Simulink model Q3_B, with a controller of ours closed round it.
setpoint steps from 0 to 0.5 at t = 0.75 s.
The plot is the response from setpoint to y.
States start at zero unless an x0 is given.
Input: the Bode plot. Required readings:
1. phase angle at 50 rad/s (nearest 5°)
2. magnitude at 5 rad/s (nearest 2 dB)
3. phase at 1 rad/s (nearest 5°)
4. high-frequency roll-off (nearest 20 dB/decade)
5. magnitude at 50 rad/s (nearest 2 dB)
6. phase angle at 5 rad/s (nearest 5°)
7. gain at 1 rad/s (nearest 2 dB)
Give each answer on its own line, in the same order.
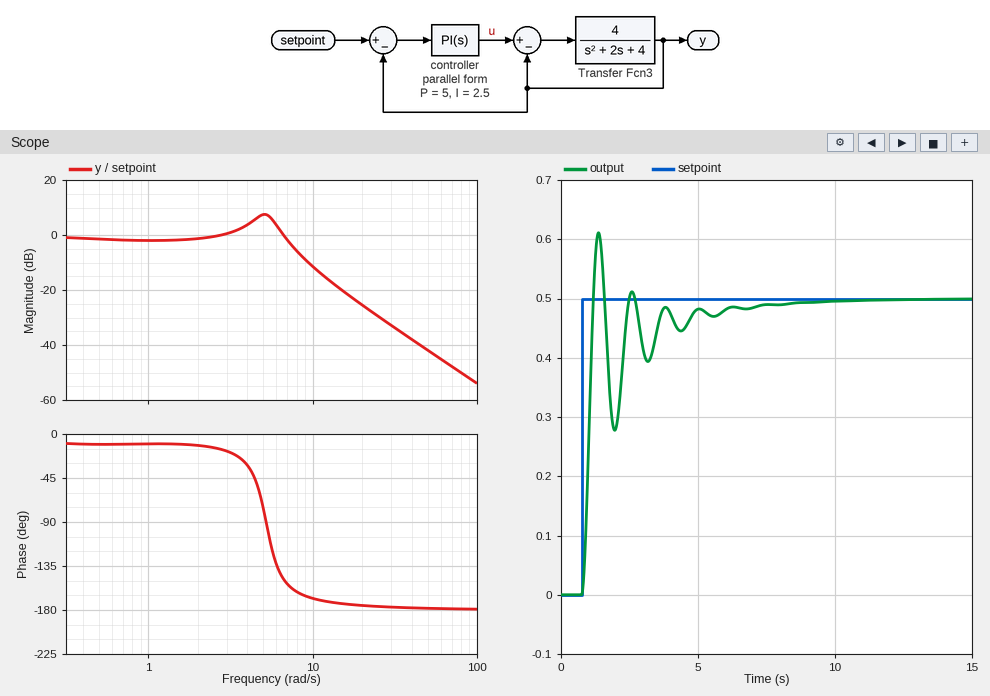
-180°
8 dB
-10°
-40 dB/decade
-42 dB
-75°
-2 dB
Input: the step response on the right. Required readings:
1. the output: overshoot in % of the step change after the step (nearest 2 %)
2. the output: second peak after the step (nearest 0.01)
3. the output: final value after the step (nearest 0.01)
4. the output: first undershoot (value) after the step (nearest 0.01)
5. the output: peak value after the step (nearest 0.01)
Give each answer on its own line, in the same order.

22 %
0.51
0.50
0.28
0.61
